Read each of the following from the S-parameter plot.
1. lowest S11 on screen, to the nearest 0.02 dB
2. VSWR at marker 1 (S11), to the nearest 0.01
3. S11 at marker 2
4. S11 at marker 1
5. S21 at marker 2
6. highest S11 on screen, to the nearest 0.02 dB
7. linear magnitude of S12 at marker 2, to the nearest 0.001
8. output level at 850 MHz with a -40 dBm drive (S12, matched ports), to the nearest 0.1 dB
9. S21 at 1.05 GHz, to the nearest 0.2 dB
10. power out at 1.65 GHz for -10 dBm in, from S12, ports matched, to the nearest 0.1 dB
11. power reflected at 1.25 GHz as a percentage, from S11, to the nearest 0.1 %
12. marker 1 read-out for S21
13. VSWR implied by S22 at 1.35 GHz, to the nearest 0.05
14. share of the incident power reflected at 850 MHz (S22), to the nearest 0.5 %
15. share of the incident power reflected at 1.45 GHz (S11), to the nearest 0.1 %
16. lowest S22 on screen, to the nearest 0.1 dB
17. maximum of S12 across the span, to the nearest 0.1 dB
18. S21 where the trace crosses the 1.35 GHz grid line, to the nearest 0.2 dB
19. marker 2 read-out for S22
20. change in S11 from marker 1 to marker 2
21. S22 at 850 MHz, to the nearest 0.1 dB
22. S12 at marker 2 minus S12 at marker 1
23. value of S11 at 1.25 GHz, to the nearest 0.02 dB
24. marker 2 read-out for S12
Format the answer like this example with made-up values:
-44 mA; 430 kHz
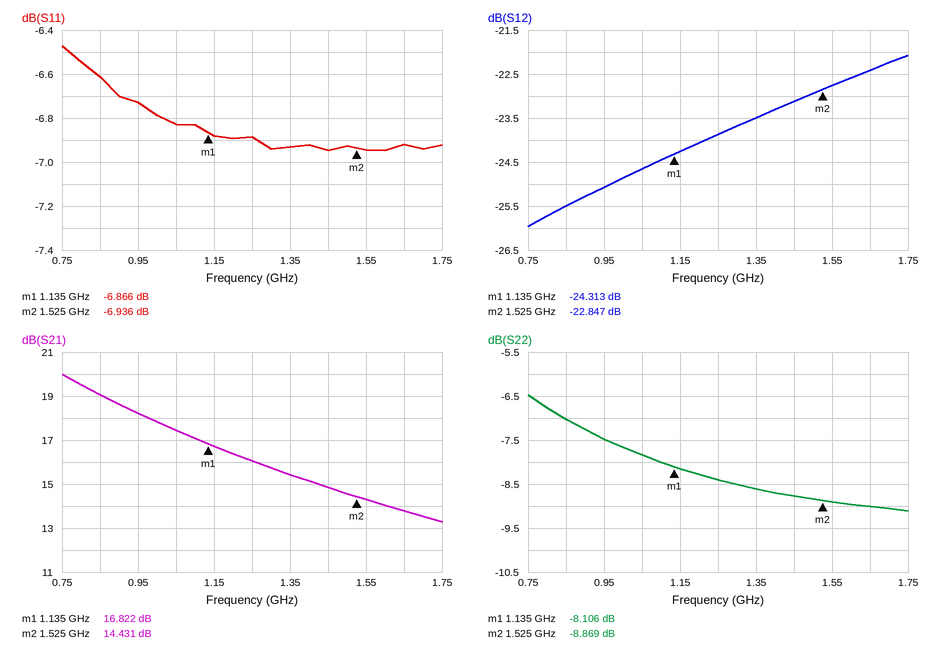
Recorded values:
-6.94 dB; 2.66; -6.936 dB; -6.866 dB; 14.431 dB; -6.48 dB; 0.072; -65.5 dBm; 17.4 dB; -32.4 dBm; 20.5 %; 16.822 dB; 2.20; 20.0 %; 20.2 %; -9.1 dB; -22.1 dB; 15.4 dB; -8.869 dB; -0.070 dB; -7.0 dB; 1.466 dB; -6.88 dB; -22.847 dB
